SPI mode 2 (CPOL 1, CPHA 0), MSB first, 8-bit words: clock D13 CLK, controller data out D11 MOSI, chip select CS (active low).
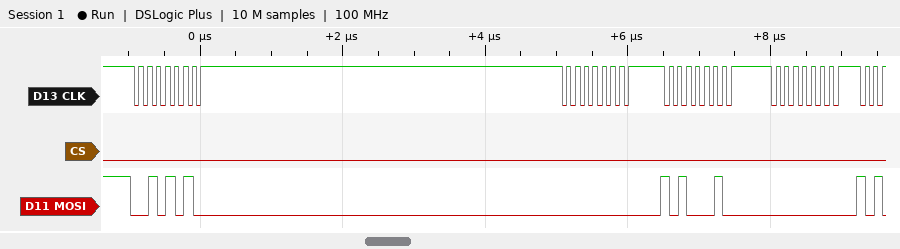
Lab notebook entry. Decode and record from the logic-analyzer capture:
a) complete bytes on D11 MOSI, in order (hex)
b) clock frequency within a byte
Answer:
2A 00 A2 00
8 MHz
